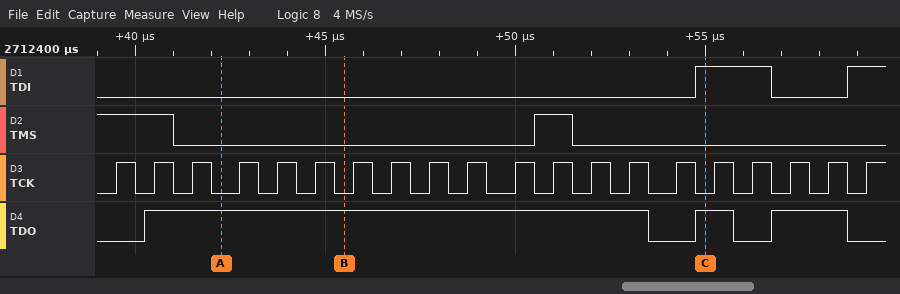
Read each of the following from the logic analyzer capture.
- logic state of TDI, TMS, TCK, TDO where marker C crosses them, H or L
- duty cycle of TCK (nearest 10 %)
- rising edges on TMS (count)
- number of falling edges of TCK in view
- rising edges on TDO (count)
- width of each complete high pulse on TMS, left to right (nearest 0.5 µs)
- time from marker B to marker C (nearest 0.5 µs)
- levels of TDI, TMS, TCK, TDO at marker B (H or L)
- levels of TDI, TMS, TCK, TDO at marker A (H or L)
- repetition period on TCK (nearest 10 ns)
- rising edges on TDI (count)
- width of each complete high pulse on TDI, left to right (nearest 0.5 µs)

TDI=H, TMS=L, TCK=L, TDO=H
50 %
1
19
3
1 µs
9.5 µs
TDI=L, TMS=L, TCK=L, TDO=H
TDI=L, TMS=L, TCK=L, TDO=H
1040 ns
2
2 µs
